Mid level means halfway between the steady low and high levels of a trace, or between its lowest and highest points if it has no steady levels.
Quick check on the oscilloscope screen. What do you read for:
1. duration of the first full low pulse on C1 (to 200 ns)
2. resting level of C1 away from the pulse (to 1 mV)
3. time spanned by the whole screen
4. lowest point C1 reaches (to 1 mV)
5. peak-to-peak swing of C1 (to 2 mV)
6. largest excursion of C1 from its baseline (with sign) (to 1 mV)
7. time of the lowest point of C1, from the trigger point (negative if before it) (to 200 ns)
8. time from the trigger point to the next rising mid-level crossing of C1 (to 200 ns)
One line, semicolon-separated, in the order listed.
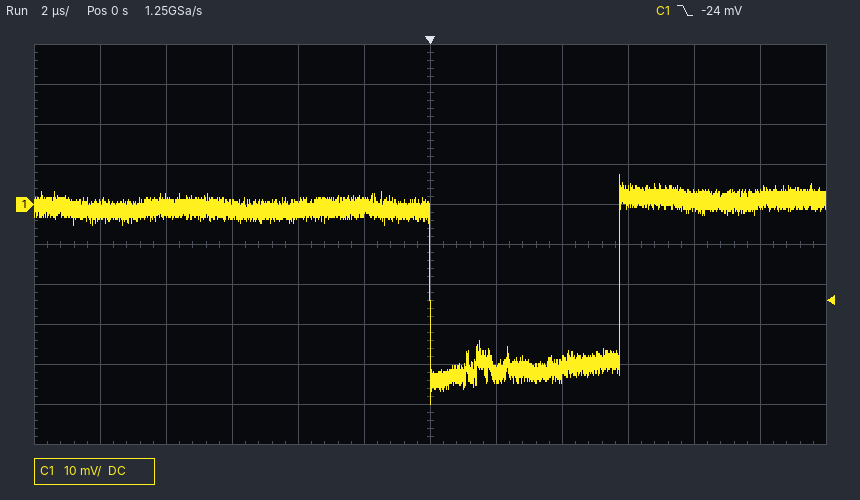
5.8 µs; -1 mV; 24 µs; -50 mV; 58 mV; -49 mV; 0.0 µs; 5.8 µs
